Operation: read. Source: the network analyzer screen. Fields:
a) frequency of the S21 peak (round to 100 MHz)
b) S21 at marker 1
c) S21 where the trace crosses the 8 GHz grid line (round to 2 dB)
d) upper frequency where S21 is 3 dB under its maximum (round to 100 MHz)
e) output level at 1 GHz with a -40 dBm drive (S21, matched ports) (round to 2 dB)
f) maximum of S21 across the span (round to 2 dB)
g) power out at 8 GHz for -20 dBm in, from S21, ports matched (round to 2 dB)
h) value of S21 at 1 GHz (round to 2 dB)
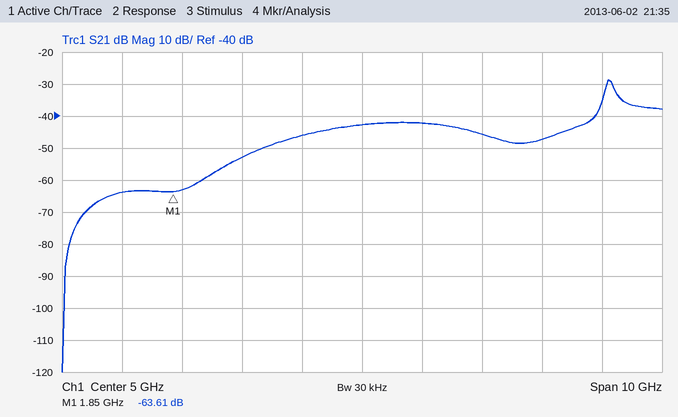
9.1 GHz
-63.61 dB
-48 dB
9.2 GHz
-104 dBm
-28 dB
-68 dBm
-64 dB
